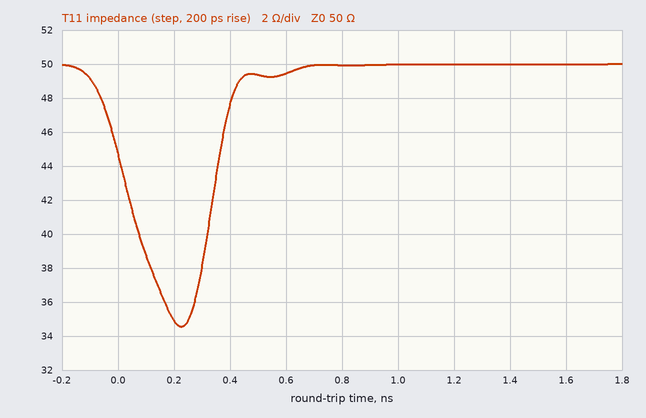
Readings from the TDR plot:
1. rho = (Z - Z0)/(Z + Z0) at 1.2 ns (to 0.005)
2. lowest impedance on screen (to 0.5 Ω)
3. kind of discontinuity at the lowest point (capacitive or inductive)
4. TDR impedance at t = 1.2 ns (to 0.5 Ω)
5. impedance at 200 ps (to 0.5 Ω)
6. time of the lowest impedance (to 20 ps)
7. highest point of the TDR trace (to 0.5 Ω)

0.000
34.5 Ω
capacitive
50.0 Ω
35.0 Ω
220 ps
50.0 Ω
